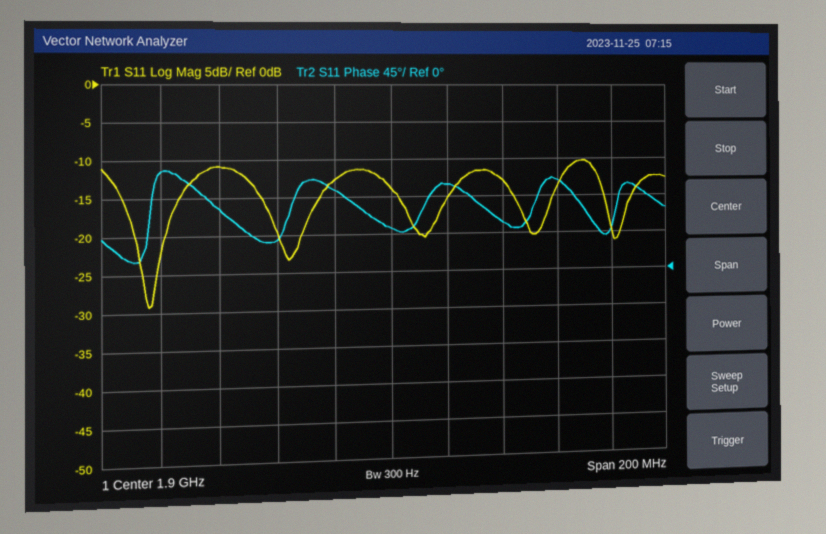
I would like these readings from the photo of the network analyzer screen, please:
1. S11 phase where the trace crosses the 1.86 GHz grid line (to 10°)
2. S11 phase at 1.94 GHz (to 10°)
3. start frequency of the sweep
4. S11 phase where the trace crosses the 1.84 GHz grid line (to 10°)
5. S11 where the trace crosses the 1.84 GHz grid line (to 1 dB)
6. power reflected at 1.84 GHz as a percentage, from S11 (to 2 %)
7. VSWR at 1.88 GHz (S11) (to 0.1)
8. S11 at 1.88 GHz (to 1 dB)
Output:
40°
60°
1.8 GHz
80°
-11 dB
8 %
1.6
-13 dB
